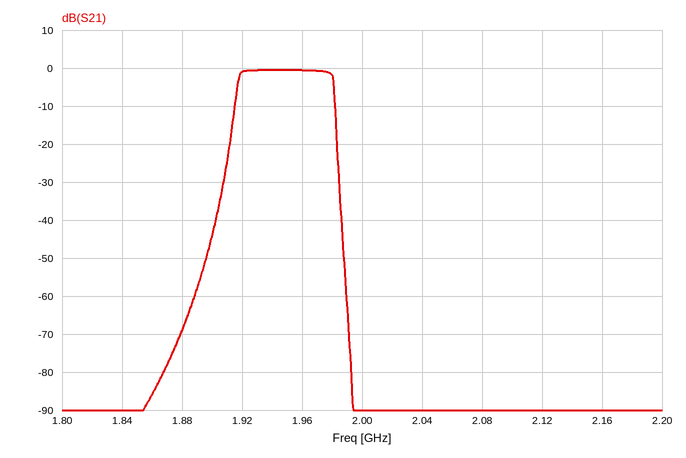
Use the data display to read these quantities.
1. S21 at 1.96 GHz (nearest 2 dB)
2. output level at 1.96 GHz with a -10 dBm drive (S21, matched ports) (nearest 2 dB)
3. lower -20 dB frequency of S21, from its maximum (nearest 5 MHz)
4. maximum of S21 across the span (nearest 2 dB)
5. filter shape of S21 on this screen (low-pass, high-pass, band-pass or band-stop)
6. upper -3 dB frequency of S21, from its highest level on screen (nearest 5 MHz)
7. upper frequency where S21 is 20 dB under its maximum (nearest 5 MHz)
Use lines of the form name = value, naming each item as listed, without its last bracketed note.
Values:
S21 at 1.96 GHz = 0 dB
output level at 1.96 GHz with a -10 dBm drive (S21, matched ports) = -10 dBm
lower -20 dB frequency of S21, from its maximum = 1.910 GHz
maximum of S21 across the span = 0 dB
filter shape of S21 on this screen = band-pass
upper -3 dB frequency of S21, from its highest level on screen = 1.980 GHz
upper frequency where S21 is 20 dB under its maximum = 1.985 GHz
